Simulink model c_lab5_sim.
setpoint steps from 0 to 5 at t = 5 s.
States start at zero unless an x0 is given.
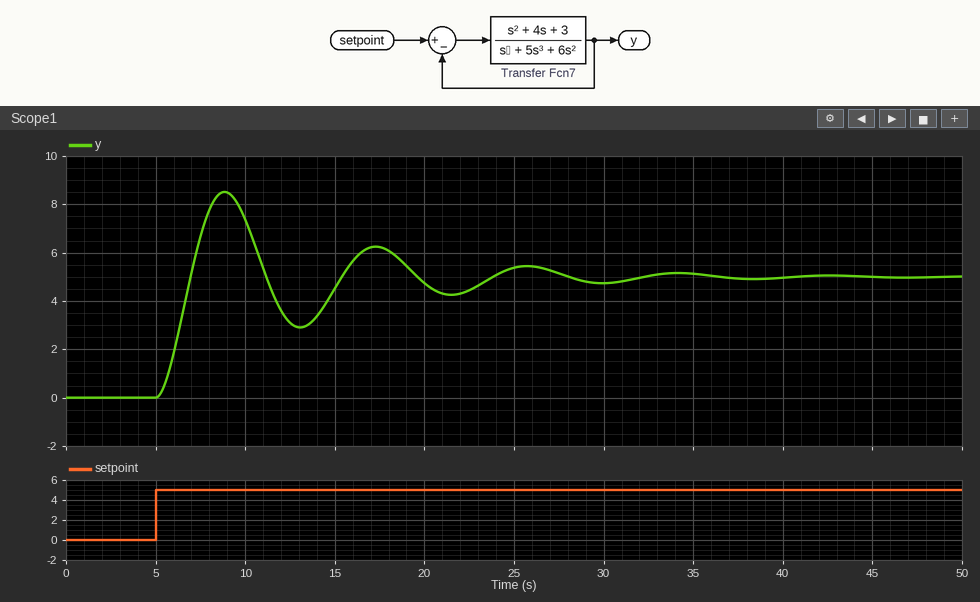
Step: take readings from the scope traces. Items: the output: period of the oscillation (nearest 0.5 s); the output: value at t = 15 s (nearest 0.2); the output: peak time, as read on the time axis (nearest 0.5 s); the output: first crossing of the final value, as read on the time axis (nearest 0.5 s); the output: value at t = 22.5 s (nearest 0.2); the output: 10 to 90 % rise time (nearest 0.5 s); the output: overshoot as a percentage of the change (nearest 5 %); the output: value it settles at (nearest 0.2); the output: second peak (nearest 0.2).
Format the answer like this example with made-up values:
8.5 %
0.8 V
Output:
8.5 s
4.6
9.0 s
7.0 s
4.4
1.5 s
70 %
5.0
6.2
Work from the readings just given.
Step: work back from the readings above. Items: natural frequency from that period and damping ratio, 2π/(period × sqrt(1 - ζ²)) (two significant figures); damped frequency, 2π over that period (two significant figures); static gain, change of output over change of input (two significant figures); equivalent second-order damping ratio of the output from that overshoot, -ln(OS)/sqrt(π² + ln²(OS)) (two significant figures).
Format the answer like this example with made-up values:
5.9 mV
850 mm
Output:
0.74 rad/s
0.74 rad/s
1.0
0.11
